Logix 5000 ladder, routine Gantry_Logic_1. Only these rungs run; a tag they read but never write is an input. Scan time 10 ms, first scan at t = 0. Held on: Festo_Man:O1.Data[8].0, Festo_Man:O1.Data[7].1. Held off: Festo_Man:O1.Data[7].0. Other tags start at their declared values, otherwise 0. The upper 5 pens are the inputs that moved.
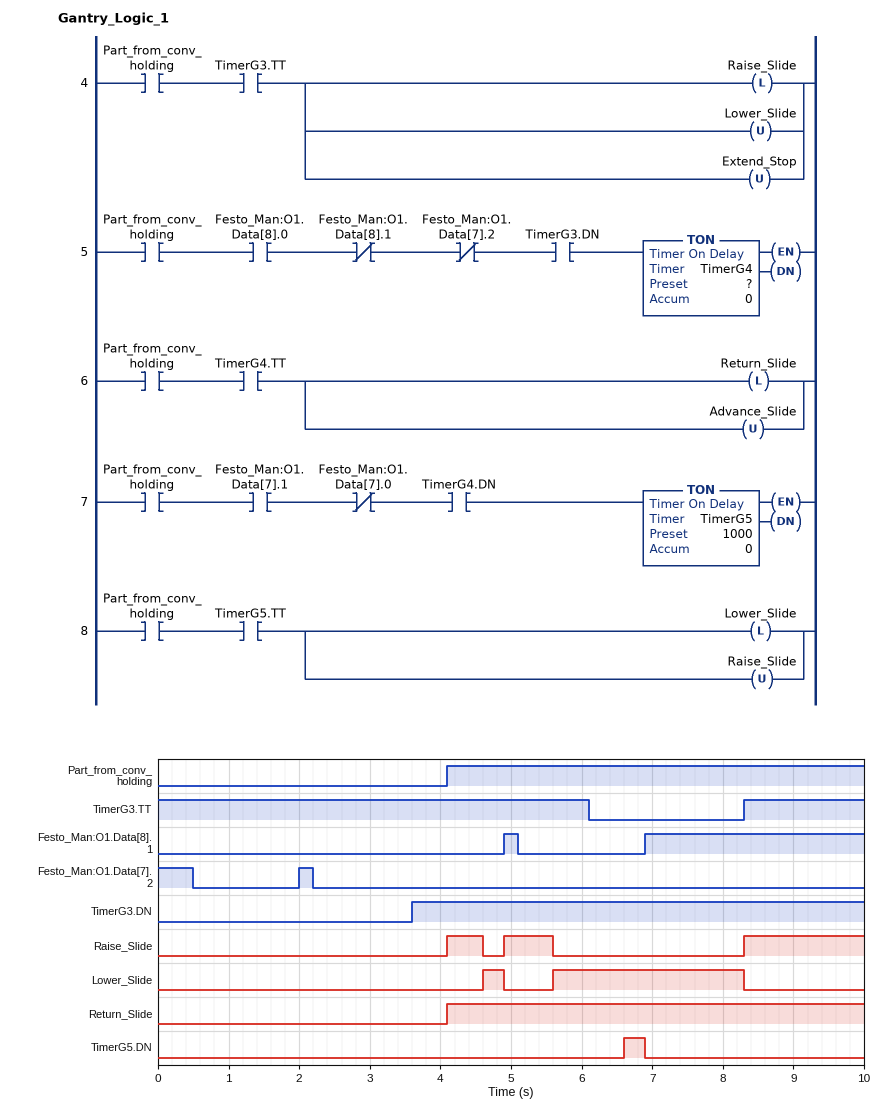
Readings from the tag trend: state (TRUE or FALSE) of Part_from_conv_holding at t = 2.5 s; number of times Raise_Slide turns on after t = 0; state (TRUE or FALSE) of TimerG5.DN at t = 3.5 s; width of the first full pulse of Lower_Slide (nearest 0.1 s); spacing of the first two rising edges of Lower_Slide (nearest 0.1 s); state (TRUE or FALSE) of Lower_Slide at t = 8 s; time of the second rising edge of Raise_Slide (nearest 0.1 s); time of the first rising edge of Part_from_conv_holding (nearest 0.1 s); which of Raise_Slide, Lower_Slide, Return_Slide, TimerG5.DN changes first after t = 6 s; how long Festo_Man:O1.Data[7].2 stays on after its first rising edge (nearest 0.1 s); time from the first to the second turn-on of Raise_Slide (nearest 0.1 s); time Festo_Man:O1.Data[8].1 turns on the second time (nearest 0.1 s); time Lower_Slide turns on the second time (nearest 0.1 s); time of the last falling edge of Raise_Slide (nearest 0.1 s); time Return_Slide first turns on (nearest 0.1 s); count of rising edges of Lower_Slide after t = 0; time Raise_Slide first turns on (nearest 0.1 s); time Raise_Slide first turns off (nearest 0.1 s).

FALSE
3
FALSE
0.3 s
1.0 s
TRUE
4.9 s
4.1 s
TimerG5.DN
0.2 s
0.8 s
6.9 s
5.6 s
5.6 s
4.1 s
2
4.1 s
4.6 s
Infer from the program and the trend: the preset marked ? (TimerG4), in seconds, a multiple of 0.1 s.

0.5 s
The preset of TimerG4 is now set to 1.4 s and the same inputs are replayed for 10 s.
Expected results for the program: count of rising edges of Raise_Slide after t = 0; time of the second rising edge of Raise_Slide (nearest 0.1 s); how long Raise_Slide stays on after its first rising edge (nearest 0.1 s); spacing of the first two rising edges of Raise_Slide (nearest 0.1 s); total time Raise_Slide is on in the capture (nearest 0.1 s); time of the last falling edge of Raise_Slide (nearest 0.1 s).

2
8.3 s
2.4 s
4.2 s
4.1 s
6.5 s
